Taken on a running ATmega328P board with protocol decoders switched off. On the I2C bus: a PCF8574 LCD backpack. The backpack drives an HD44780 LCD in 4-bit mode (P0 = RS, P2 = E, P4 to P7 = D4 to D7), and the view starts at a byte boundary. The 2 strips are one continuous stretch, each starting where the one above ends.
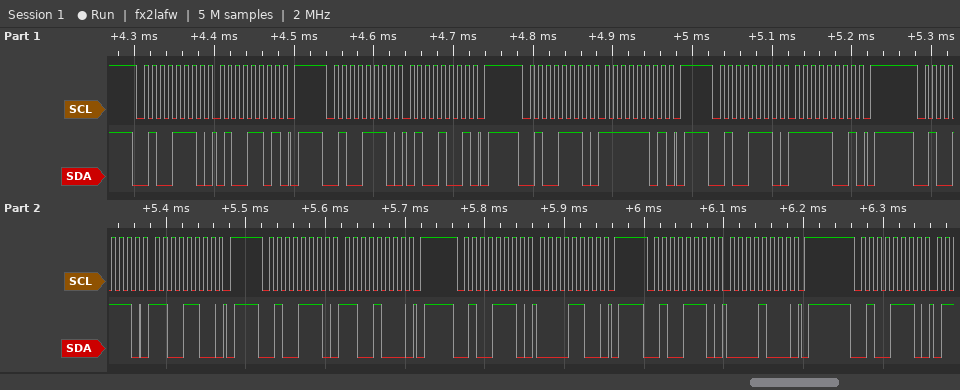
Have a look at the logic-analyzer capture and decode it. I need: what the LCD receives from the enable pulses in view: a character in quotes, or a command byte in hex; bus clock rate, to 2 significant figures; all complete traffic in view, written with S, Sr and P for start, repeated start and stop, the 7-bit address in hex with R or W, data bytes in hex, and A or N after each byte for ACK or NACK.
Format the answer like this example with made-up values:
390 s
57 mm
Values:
'O' 0xC0
100 kHz
S 27W A 4D A P S 27W A 49 A P S 27W A FD A P S 27W A F9 A P S 27W A CC A P S 27W A C8 A P S 27W A 0C A P S 27W A 08 A P S 27W A
